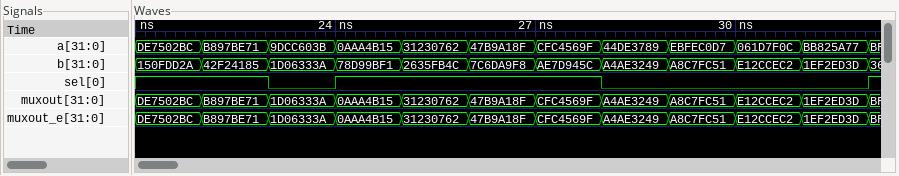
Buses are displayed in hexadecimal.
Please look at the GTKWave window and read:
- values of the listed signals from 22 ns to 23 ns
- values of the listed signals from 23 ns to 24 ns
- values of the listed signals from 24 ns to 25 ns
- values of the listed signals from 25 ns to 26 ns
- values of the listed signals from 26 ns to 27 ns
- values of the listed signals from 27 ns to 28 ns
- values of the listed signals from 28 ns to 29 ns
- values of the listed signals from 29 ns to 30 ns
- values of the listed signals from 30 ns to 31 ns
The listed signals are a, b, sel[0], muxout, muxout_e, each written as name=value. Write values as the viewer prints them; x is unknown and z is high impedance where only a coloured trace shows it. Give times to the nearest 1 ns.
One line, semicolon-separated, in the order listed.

a=B897BE71, b=42F24185, sel[0]=1, muxout=B897BE71, muxout_e=B897BE71; a=9DCC603B, b=1D06333A, sel[0]=0, muxout=1D06333A, muxout_e=1D06333A; a=0AAA4B15, b=78D99BF1, sel[0]=1, muxout=0AAA4B15, muxout_e=0AAA4B15; a=31230762, b=2635FB4C, sel[0]=1, muxout=31230762, muxout_e=31230762; a=47B9A18F, b=7C6DA9F8, sel[0]=1, muxout=47B9A18F, muxout_e=47B9A18F; a=CFC4569F, b=AE7D945C, sel[0]=1, muxout=CFC4569F, muxout_e=CFC4569F; a=44DE3789, b=A4AE3249, sel[0]=0, muxout=A4AE3249, muxout_e=A4AE3249; a=EBFEC0D7, b=A8C7FC51, sel[0]=0, muxout=A8C7FC51, muxout_e=A8C7FC51; a=061D7F0C, b=E12CCEC2, sel[0]=0, muxout=E12CCEC2, muxout_e=E12CCEC2
